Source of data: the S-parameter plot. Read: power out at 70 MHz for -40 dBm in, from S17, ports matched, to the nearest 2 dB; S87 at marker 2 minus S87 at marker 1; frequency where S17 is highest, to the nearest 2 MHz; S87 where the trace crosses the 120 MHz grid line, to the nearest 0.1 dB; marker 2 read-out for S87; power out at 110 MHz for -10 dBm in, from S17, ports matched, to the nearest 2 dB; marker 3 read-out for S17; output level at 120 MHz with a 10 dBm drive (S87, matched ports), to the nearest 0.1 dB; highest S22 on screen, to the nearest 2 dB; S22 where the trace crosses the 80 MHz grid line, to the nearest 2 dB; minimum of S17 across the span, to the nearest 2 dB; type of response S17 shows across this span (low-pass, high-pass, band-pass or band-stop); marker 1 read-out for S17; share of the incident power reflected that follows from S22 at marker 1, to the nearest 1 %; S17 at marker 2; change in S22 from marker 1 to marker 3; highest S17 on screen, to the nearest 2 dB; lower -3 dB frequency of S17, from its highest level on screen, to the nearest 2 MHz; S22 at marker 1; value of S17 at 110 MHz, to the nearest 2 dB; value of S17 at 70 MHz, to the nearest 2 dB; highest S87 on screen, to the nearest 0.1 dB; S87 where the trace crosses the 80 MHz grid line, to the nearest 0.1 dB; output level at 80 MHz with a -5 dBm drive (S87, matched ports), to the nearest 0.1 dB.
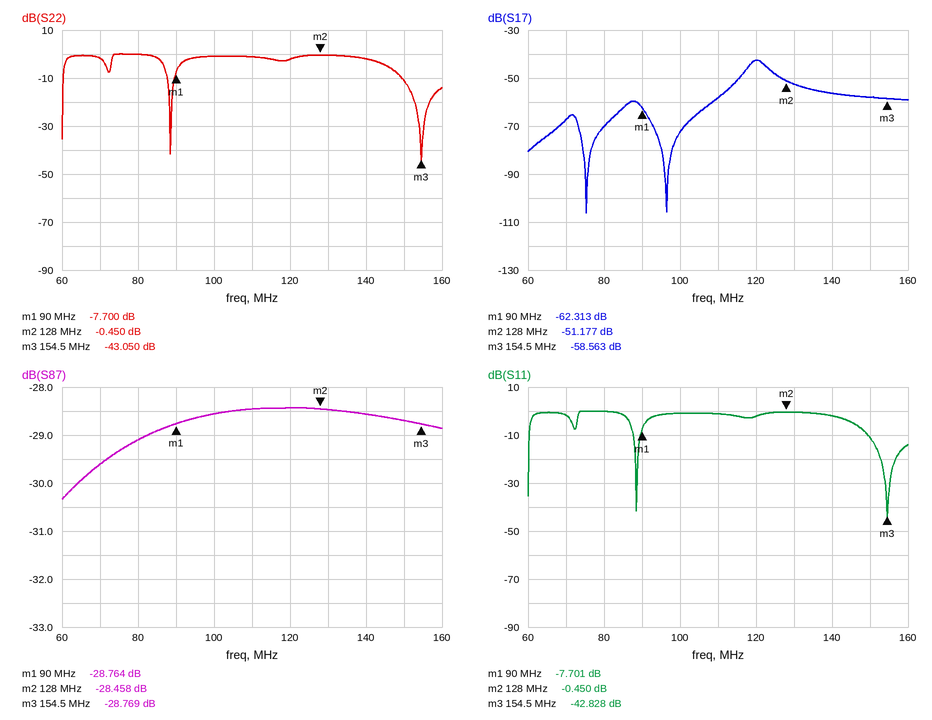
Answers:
-108 dBm
0.306 dB
120 MHz
-28.4 dB
-28.458 dB
-68 dBm
-58.563 dB
-18.4 dBm
0 dB
0 dB
-106 dB
band-pass
-62.313 dB
17 %
-51.177 dB
-35.350 dB
-42 dB
118 MHz
-7.700 dB
-58 dB
-68 dB
-28.4 dB
-29.1 dB
-34.1 dBm
